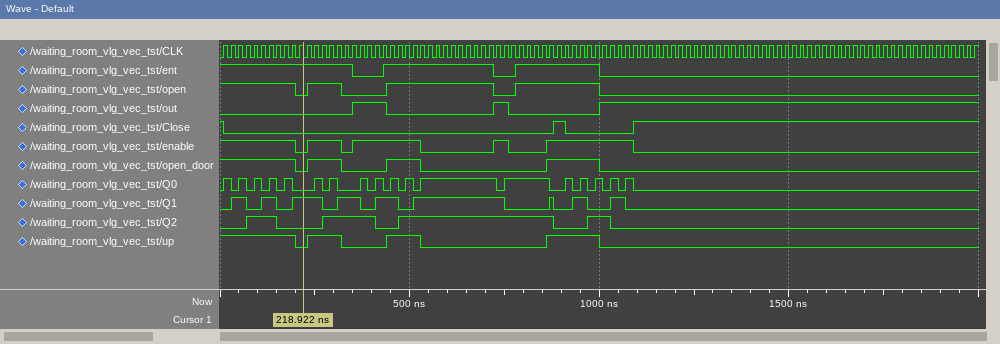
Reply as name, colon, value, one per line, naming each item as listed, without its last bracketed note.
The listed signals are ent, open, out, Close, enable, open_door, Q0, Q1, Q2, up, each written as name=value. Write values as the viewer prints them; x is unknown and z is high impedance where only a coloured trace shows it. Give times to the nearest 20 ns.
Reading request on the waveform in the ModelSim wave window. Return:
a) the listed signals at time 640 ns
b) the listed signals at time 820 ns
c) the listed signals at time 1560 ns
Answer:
the listed signals at time 640 ns: ent=1, open=1, out=0, Close=0, enable=0, open_door=0, Q0=1, Q1=1, Q2=1, up=0
the listed signals at time 820 ns: ent=1, open=1, out=0, Close=0, enable=0, open_door=0, Q0=1, Q1=0, Q2=1, up=0
the listed signals at time 1560 ns: ent=0, open=0, out=1, Close=1, enable=0, open_door=0, Q0=0, Q1=0, Q2=0, up=0
